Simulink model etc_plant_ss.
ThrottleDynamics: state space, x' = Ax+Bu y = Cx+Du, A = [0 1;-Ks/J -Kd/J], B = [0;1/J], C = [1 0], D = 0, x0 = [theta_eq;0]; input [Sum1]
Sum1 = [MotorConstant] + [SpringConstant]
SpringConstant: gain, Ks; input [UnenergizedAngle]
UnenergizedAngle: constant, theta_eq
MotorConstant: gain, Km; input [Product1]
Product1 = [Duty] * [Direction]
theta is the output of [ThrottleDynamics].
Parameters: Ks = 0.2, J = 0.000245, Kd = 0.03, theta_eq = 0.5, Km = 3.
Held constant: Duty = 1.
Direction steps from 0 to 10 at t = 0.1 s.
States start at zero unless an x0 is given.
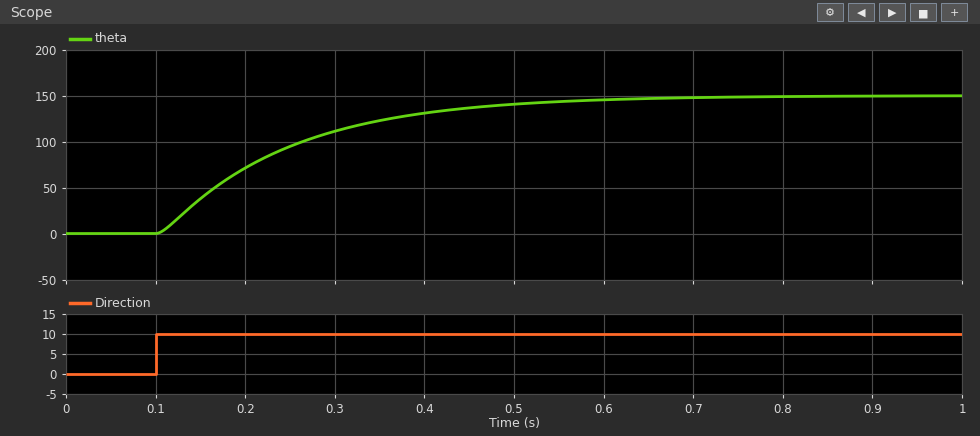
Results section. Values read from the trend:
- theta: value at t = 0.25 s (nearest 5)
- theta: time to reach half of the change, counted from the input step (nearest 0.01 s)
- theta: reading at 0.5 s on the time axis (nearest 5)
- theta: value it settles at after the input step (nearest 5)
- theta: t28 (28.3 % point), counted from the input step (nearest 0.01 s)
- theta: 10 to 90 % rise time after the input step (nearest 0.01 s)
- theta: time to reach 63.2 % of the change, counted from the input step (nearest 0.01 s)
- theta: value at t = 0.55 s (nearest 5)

95
0.11 s
140
150
0.06 s
0.31 s
0.15 s
145
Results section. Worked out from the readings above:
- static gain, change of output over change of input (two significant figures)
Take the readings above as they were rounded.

15
